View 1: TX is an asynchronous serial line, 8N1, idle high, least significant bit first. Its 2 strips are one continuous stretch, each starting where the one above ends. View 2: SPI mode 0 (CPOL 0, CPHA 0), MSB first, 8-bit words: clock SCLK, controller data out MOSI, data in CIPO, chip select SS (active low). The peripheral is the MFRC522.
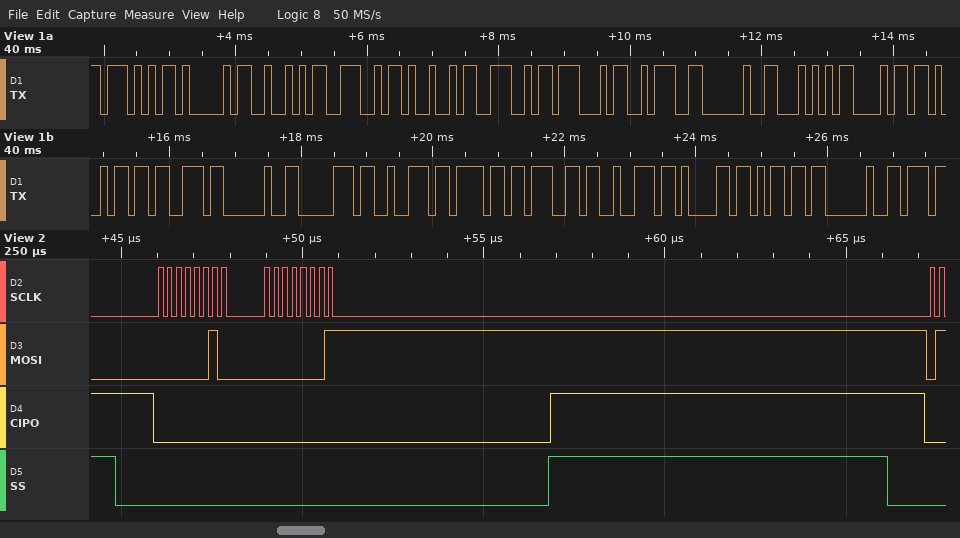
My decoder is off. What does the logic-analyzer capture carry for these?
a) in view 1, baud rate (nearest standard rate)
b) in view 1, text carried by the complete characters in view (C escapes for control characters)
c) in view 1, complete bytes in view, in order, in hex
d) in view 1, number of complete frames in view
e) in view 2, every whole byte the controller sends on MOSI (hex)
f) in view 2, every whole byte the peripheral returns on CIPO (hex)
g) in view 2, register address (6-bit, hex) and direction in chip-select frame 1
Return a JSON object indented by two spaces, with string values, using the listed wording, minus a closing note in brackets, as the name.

{
  "in view 1, baud rate": "9600 baud",
  "in view 1, text carried by the complete characters in view": "\"WARNING: This program \"",
  "in view 1, complete bytes in view, in order, in hex": "57 41 52 4E 49 4E 47 3A 20 54 68 69 73 20 70 72 6F 67 72 61 6D 20",
  "in view 1, number of complete frames in view": "22",
  "in view 2, every whole byte the controller sends on MOSI": "02 01",
  "in view 2, every whole byte the peripheral returns on CIPO": "00 00",
  "in view 2, register address (6-bit, hex) and direction in chip-select frame 1": "0x01 write"
}
